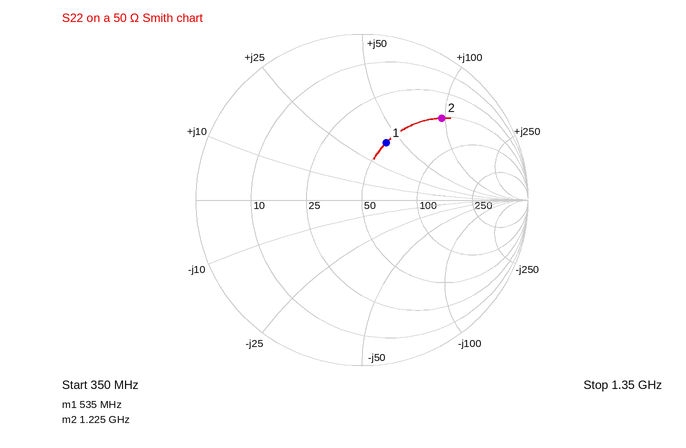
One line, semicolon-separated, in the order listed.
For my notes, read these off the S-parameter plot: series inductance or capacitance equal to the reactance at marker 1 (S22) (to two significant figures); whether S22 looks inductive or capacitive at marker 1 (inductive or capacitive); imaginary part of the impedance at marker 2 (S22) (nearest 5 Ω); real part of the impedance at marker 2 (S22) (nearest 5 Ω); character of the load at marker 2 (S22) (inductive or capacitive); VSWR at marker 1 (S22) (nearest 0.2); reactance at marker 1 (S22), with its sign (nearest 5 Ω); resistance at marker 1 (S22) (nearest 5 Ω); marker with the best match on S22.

12 nH; inductive; +95 Ω; 50 Ω; inductive; 2.2; +40 Ω; 50 Ω; marker 1
